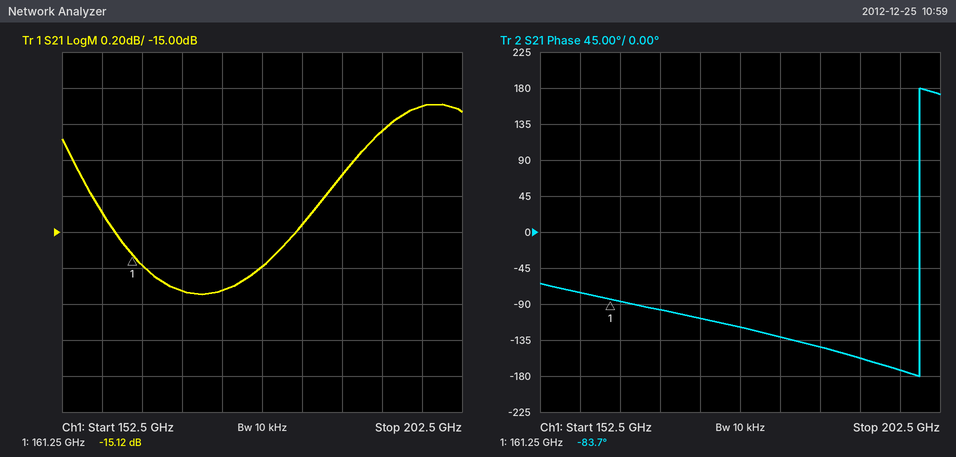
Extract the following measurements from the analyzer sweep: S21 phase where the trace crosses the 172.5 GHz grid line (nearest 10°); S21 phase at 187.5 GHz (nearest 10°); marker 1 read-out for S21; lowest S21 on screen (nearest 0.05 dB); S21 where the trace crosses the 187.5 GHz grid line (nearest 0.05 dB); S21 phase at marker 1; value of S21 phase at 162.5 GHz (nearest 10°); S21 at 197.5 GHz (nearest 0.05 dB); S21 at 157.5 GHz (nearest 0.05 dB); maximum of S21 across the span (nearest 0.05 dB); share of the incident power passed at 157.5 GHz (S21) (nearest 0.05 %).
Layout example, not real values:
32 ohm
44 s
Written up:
-110°
-140°
-15.12 dB
-15.35 dB
-14.70 dB
-83.7°
-90°
-14.30 dB
-14.90 dB
-14.30 dB
3.25 %
